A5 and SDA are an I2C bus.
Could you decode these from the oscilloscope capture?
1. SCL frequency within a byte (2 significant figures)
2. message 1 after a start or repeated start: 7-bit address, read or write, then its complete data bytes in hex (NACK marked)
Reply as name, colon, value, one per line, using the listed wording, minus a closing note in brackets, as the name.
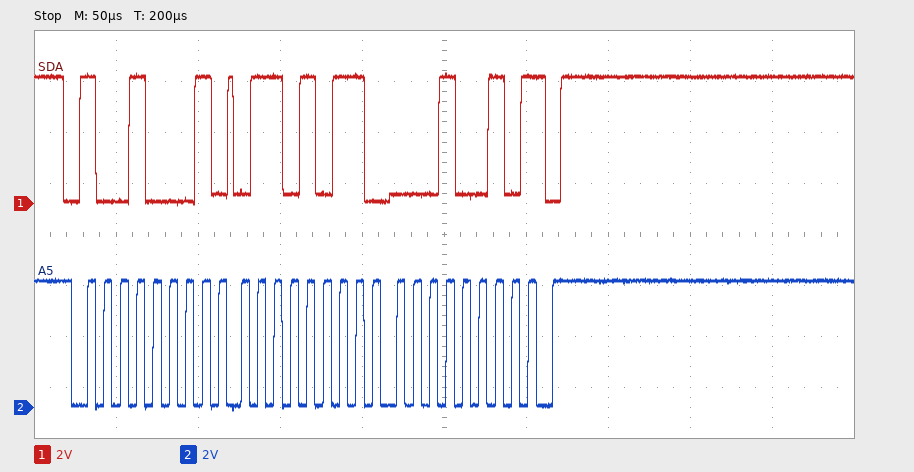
SCL frequency within a byte: 100 kHz
message 1 after a start or repeated start: 7-bit address, read or write, then its complete data bytes in hex: 0x48 read: 6B 12 NACK
